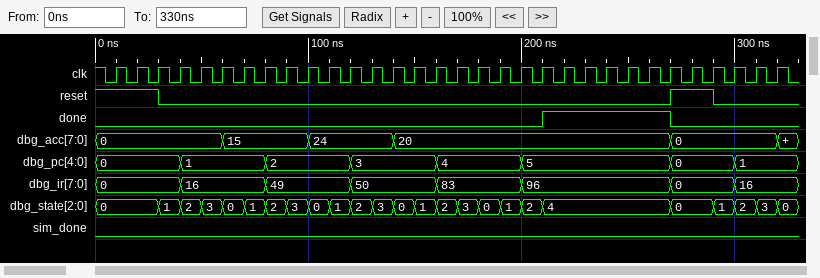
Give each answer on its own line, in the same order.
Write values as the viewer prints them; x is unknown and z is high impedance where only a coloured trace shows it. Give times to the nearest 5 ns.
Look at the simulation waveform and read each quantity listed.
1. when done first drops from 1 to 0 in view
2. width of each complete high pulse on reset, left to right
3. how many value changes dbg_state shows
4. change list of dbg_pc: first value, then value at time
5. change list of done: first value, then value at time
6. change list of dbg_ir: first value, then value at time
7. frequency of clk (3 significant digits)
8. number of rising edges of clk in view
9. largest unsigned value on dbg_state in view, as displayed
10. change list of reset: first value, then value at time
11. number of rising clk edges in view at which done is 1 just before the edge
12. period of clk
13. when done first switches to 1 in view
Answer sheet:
270 ns
20 ns
24
0, 1 at 40 ns, 2 at 80 ns, 3 at 120 ns, 4 at 160 ns, 5 at 200 ns, 0 at 270 ns, 1 at 300 ns
0, 1 at 210 ns, 0 at 270 ns
0, 16 at 40 ns, 49 at 80 ns, 50 at 120 ns, 83 at 160 ns, 96 at 200 ns, 0 at 270 ns, 16 at 300 ns
100 MHz
32
4
1, 0 at 30 ns, 1 at 270 ns, 0 at 290 ns
6
10 ns
210 ns
